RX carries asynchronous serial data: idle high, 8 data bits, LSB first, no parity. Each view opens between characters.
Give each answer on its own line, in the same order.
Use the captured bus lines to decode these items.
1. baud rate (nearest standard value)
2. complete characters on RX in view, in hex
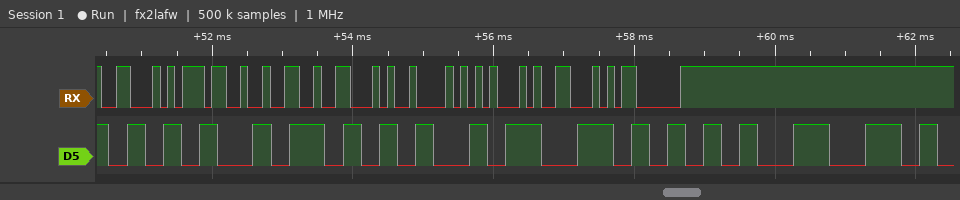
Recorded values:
9600 baud
46, 37, 32, 46, 42, 45, 46, 03
